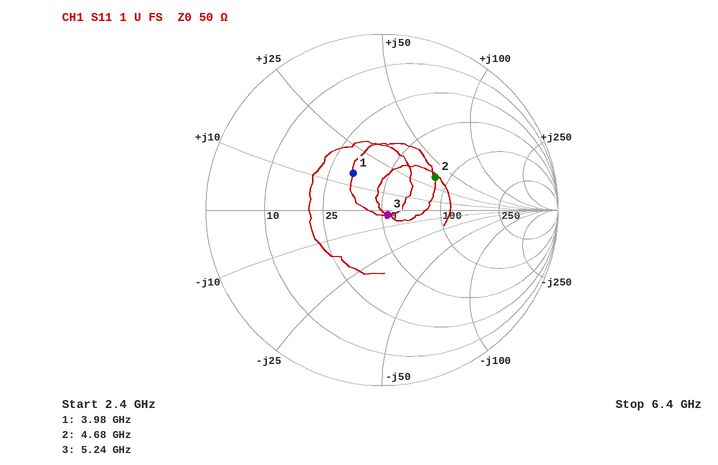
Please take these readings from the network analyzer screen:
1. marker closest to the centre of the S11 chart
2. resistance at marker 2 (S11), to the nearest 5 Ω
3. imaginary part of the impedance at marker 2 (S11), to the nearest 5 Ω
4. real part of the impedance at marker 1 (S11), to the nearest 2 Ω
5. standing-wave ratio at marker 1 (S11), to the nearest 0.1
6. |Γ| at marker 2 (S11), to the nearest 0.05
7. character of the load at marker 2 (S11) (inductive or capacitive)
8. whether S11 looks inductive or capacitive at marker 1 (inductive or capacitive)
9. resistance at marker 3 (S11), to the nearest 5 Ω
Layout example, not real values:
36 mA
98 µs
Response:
marker 3
85 Ω
+35 Ω
34 Ω
1.7
0.35
inductive
inductive
55 Ω
